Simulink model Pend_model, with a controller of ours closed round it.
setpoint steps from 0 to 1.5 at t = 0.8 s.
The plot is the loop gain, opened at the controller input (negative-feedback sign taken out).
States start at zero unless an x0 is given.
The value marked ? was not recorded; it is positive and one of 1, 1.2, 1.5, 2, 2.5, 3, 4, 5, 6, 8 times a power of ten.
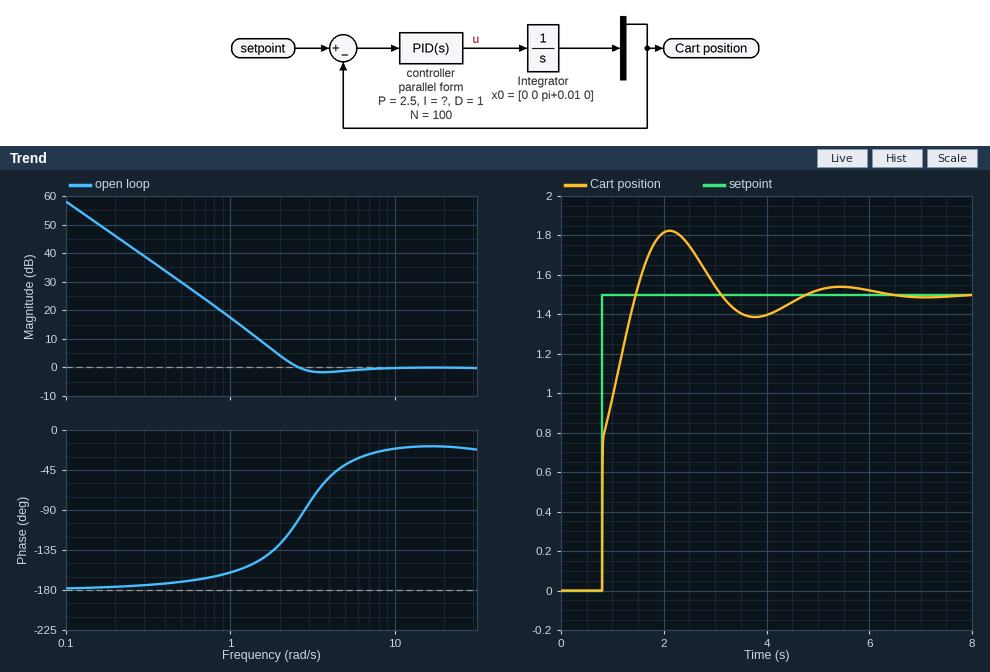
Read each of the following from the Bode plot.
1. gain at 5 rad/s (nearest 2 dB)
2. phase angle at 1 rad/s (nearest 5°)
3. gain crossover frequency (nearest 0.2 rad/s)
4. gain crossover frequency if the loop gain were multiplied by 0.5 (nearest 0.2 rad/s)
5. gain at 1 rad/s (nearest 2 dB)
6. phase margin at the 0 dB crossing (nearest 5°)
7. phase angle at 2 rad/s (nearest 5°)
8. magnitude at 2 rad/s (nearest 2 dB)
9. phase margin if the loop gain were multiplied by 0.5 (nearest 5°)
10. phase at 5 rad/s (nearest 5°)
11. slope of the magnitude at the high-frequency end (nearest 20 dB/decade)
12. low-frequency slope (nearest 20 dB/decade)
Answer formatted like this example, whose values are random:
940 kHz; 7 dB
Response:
-2 dB; -160°; 2.6 rad/s; 1.8 rad/s; 18 dB; 80°; -130°; 4 dB; 45°; -40°; 0 dB/decade; -40 dB/decade
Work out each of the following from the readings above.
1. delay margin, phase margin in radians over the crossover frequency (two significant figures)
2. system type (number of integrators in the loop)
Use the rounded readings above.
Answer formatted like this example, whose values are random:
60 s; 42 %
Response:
0.54 s; 2
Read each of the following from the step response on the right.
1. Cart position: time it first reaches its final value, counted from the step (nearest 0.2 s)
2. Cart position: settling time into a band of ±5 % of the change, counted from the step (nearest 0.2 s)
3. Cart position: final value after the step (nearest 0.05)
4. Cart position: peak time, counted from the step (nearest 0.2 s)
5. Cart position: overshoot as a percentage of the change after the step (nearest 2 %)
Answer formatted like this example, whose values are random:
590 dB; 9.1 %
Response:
0.6 s; 3.4 s; 1.50; 1.4 s; 22 %
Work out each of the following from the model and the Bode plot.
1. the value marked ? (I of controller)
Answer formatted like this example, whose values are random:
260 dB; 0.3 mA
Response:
8
